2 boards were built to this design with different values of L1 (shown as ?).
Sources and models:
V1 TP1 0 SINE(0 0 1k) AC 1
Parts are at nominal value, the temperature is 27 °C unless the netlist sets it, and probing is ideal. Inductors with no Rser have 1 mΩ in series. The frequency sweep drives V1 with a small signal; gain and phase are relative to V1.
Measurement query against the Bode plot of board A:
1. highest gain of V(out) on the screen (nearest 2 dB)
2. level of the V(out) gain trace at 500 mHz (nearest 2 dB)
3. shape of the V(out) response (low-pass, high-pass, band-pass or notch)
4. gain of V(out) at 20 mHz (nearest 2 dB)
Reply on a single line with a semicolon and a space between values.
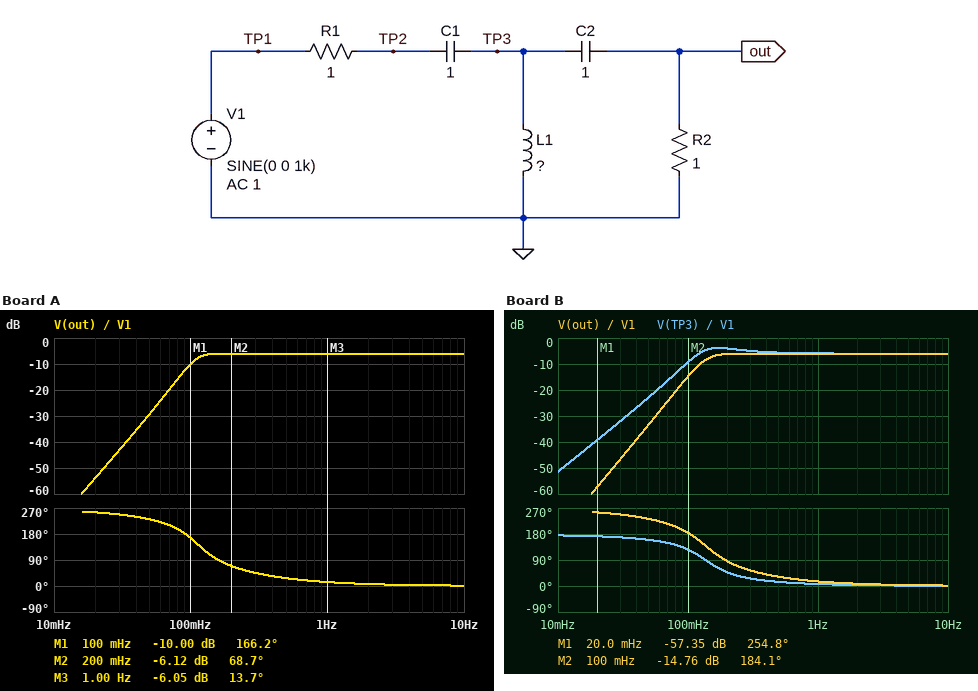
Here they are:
-6 dB; -6 dB; high-pass; -54 dB
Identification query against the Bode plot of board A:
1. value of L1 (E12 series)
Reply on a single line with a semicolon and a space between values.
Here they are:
1 H
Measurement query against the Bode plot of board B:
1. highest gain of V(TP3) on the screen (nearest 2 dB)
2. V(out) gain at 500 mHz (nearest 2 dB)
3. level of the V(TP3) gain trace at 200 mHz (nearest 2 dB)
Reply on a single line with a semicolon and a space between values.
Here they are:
-4 dB; -6 dB; -4 dB
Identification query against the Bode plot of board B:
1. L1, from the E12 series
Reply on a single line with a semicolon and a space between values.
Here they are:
680 mH
